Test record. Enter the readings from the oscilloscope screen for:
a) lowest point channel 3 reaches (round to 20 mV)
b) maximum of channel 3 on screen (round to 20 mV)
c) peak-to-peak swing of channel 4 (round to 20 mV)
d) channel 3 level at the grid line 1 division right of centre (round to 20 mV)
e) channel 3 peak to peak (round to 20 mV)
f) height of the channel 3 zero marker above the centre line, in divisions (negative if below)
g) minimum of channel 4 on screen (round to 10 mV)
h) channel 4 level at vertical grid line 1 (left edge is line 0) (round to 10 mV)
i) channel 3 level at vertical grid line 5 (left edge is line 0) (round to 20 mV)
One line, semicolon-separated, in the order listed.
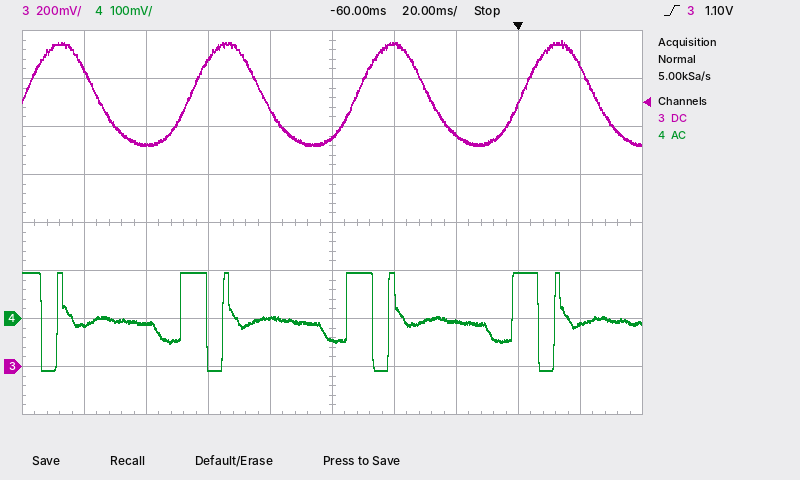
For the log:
920 mV; 1.36 V; 200 mV; 1.34 V; 440 mV; -3.0 div; -110 mV; -10 mV; 960 mV
